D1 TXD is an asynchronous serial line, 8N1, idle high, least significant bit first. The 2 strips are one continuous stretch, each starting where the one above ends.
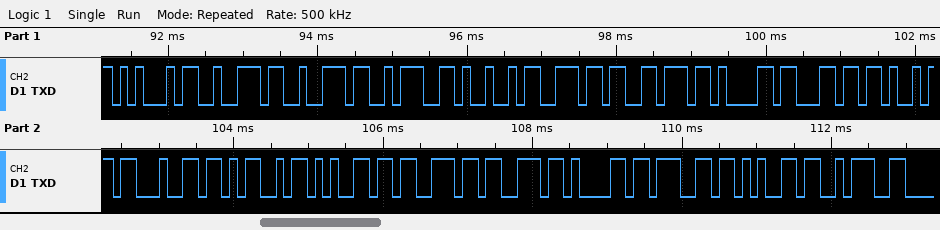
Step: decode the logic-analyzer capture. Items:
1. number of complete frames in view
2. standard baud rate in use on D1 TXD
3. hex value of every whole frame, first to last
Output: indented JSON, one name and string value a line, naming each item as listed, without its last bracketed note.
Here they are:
{
  "number of complete frames in view": "19",
  "standard baud rate in use on D1 TXD": "9600 baud",
  "hex value of every whole frame, first to last": "45 72 72 3A 49 6E 76 61 6C 69 64 4D 65 73 73 61 67 65 3A"
}
